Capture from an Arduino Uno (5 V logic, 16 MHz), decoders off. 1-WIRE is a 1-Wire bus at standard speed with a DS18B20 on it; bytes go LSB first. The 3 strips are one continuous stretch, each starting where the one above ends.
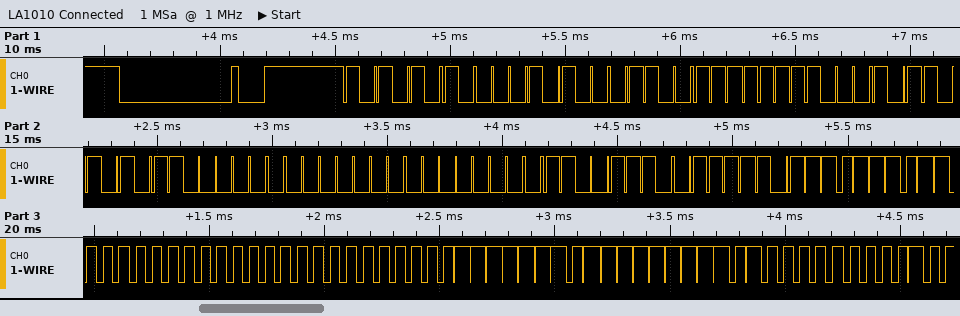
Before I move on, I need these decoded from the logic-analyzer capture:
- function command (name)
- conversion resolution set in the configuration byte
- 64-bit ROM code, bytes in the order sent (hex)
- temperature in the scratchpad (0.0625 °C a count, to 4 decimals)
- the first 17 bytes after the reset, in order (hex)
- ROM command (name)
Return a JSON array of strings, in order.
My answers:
["Read Scratchpad", "12 bits", "28 E6 1F AD 06 00 00 73", "27.6875 °C", "55 28 E6 1F AD 06 00 00 73 BE BB 01 00 00 7F FF 05", "Match ROM"]
